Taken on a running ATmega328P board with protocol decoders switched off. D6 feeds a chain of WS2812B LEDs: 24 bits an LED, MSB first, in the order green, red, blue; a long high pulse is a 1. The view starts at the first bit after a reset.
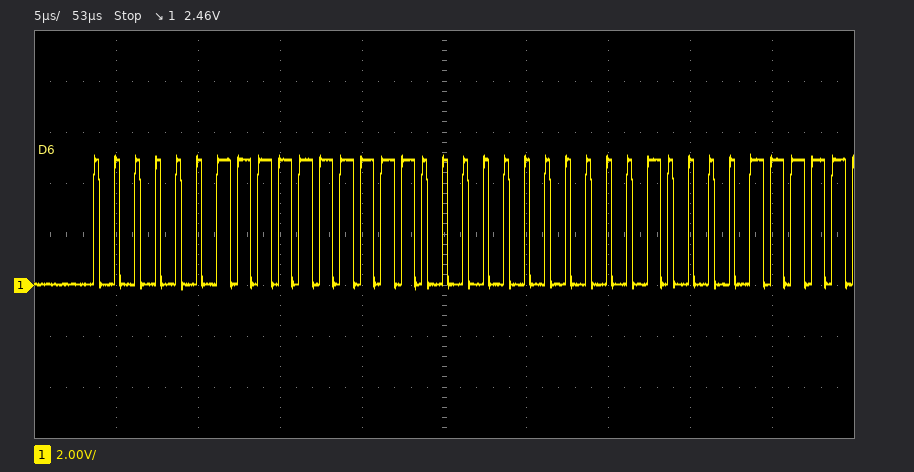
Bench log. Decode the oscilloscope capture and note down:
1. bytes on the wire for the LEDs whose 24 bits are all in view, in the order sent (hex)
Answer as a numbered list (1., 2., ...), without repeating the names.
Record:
1. 03 FF 00
